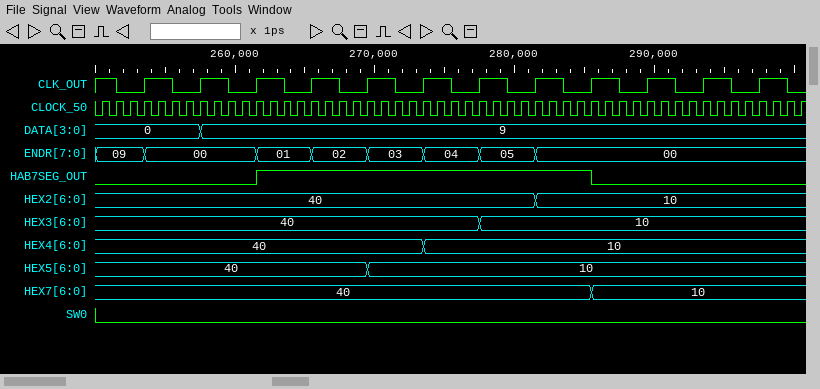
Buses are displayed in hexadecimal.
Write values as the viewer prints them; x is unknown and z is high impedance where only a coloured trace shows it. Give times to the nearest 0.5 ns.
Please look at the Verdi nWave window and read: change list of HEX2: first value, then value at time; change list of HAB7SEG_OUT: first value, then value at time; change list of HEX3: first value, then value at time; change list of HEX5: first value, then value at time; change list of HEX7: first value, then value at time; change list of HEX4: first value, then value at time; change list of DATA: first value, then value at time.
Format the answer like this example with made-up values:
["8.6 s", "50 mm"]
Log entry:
["40, 10 at 281.5 ns", "0, 1 at 261.5 ns, 0 at 285.5 ns", "40, 10 at 277.5 ns", "40, 10 at 269.5 ns", "40, 10 at 285.5 ns", "40, 10 at 273.5 ns", "0, 9 at 257.5 ns"]
